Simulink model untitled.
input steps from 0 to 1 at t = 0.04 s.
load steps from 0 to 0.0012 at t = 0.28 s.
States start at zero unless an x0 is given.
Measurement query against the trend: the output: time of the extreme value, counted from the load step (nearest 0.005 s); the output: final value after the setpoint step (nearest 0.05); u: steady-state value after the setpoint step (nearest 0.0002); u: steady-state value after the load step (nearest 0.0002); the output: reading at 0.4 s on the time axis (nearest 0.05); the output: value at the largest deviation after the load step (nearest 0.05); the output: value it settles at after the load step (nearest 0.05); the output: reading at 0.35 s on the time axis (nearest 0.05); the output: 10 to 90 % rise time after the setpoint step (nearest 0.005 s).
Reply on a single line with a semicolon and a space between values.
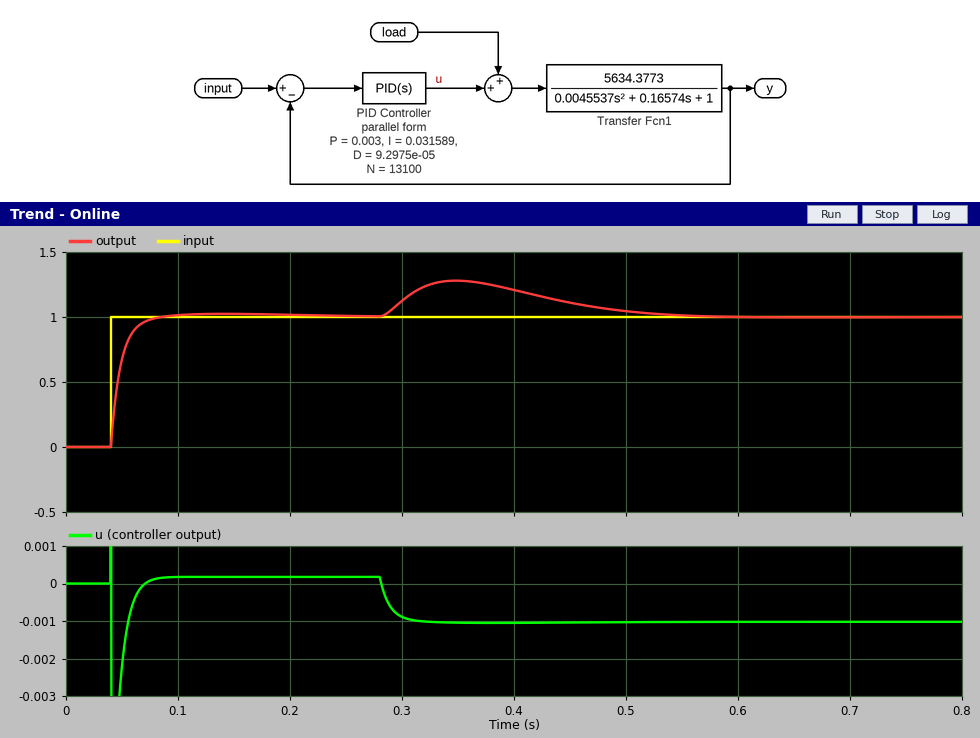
0.070 s; 1.00; 0.0002; -0.0010; 1.20; 1.30; 1.00; 1.30; 0.020 s
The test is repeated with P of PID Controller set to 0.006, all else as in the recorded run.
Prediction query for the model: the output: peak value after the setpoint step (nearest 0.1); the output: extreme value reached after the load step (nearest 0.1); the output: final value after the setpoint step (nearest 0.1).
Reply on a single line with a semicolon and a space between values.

1.1; 1.2; 1.0
